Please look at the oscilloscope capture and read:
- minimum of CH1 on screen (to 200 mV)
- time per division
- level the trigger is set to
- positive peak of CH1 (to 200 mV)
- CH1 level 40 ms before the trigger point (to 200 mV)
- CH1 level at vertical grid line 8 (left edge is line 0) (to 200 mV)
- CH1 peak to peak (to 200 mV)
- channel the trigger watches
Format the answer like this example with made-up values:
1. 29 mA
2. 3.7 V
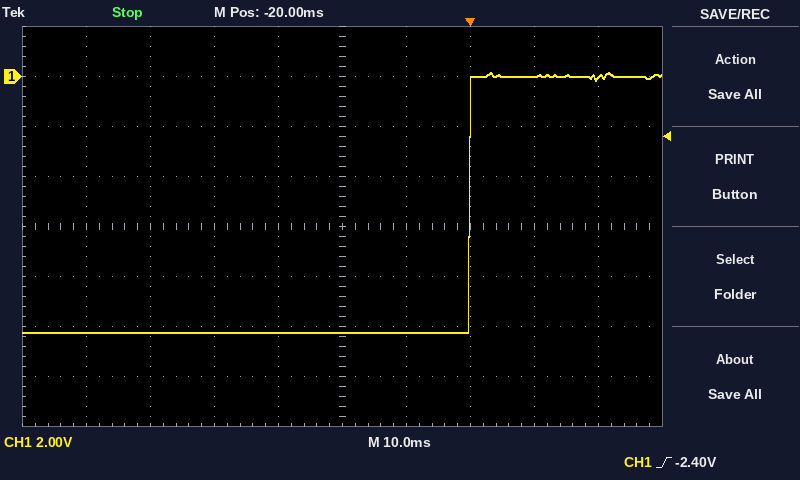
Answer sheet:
1. -10.2 V
2. 10 ms
3. -2.40 V
4. 200 mV
5. -10.2 V
6. 0.0 V
7. 10.4 V
8. CH1
